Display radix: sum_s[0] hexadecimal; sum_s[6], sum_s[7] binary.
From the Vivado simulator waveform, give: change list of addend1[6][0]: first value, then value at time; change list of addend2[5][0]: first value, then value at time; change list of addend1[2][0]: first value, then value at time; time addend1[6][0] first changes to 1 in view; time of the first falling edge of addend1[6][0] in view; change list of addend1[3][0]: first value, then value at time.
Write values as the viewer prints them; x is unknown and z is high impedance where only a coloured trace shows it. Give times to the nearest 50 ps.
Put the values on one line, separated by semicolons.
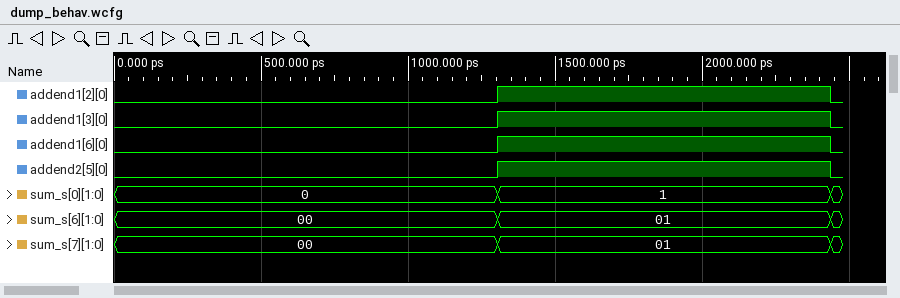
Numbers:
0, 1 at 1300 ps, 0 at 2450 ps; 0, 1 at 1300 ps, 0 at 2450 ps; 0, 1 at 1300 ps, 0 at 2450 ps; 1300 ps; 2450 ps; 0, 1 at 1300 ps, 0 at 2450 ps
